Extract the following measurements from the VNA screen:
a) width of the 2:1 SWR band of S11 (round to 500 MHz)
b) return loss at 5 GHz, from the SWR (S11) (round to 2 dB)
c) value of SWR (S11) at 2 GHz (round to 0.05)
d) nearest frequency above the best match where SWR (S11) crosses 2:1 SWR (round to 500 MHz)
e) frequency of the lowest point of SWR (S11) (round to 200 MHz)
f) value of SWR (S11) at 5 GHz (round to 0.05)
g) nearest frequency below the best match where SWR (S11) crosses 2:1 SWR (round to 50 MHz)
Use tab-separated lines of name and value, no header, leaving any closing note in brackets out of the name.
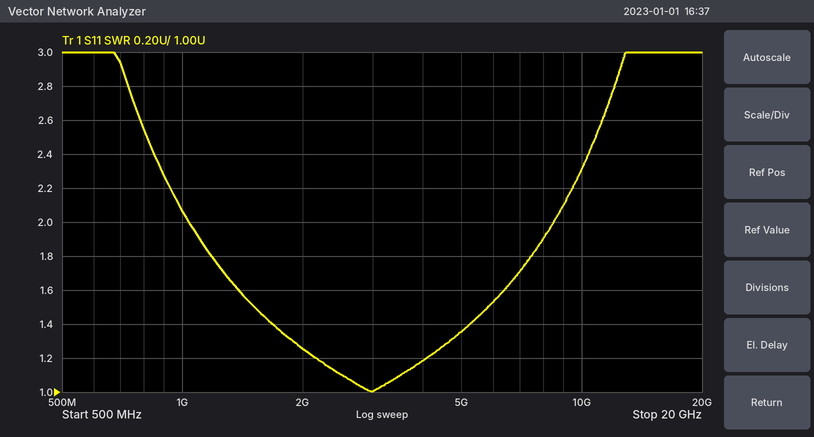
width of the 2:1 SWR band of S11	7.5 GHz
return loss at 5 GHz, from the SWR (S11)	16 dB
value of SWR (S11) at 2 GHz	1.25
nearest frequency above the best match where SWR (S11) crosses 2:1 SWR	8.5 GHz
frequency of the lowest point of SWR (S11)	3.0 GHz
value of SWR (S11) at 5 GHz	1.35
nearest frequency below the best match where SWR (S11) crosses 2:1 SWR	1.05 GHz
